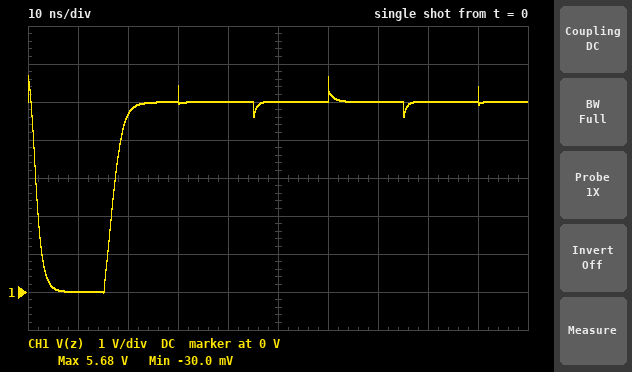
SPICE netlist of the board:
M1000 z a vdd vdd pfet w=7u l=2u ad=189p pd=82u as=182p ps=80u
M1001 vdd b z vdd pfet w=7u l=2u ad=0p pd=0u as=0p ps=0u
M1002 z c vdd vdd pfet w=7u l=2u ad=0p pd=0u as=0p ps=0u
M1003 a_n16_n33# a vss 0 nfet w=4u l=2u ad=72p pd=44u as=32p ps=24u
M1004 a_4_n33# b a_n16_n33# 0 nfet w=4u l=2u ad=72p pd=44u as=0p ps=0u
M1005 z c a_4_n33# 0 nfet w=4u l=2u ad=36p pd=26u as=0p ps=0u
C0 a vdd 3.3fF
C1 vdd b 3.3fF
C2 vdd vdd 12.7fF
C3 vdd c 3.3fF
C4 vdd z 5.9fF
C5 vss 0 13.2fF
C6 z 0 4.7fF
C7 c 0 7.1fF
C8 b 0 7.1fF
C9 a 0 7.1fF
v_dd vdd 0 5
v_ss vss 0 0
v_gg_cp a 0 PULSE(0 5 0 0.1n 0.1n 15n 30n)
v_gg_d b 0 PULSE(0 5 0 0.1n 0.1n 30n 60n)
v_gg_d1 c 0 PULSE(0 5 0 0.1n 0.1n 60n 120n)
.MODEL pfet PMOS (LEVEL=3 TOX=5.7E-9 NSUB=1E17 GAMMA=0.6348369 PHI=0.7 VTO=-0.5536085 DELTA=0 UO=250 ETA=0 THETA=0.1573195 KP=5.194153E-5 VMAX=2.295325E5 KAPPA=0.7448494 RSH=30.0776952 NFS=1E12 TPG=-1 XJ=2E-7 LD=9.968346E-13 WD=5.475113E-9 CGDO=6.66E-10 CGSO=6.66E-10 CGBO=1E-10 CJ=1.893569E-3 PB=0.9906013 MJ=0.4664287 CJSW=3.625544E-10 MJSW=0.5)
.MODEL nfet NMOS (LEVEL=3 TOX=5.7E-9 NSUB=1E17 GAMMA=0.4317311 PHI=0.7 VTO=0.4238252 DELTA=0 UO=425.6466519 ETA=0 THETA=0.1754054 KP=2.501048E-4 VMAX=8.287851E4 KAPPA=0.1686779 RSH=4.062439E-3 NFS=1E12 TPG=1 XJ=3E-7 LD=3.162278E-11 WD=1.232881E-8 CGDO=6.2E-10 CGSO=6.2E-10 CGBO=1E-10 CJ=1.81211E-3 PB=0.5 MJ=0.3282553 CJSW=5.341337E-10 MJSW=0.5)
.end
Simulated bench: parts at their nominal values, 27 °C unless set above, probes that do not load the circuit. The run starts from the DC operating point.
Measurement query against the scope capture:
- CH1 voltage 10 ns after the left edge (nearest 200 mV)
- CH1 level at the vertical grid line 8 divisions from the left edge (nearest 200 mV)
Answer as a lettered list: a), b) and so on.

a) 0 V
b) 5.0 V
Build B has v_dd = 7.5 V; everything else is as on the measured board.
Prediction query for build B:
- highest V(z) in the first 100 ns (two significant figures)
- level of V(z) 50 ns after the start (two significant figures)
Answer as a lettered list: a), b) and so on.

a) 8.2 V
b) 7.5 V
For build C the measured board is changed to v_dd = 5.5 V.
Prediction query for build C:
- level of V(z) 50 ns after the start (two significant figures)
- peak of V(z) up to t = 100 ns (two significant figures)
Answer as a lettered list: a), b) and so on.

a) 5.5 V
b) 6.2 V
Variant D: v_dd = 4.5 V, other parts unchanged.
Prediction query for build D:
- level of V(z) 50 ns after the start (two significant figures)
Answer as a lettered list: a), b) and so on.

a) 4.5 V
